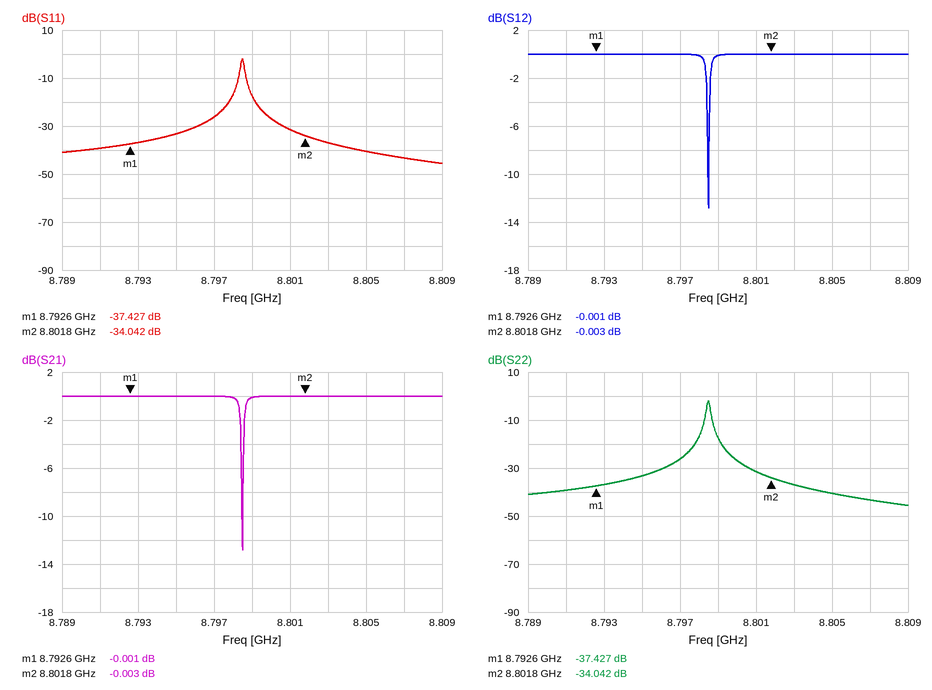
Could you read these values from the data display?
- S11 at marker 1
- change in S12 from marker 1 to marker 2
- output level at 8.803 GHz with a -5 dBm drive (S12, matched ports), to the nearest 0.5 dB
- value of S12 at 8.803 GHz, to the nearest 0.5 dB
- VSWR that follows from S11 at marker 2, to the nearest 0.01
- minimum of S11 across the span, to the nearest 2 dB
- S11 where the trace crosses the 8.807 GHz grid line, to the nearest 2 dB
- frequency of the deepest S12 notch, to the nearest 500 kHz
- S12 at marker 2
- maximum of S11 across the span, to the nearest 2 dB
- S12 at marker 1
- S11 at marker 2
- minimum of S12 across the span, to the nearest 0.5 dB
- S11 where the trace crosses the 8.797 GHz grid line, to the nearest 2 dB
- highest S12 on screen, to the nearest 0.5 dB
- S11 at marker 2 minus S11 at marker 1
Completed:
-37.427 dB
-0.002 dB
-5.0 dBm
0.0 dB
1.04
-46 dB
-44 dB
8.7985 GHz
-0.003 dB
-2 dB
-0.001 dB
-34.042 dB
-13.0 dB
-26 dB
0.0 dB
3.385 dB
